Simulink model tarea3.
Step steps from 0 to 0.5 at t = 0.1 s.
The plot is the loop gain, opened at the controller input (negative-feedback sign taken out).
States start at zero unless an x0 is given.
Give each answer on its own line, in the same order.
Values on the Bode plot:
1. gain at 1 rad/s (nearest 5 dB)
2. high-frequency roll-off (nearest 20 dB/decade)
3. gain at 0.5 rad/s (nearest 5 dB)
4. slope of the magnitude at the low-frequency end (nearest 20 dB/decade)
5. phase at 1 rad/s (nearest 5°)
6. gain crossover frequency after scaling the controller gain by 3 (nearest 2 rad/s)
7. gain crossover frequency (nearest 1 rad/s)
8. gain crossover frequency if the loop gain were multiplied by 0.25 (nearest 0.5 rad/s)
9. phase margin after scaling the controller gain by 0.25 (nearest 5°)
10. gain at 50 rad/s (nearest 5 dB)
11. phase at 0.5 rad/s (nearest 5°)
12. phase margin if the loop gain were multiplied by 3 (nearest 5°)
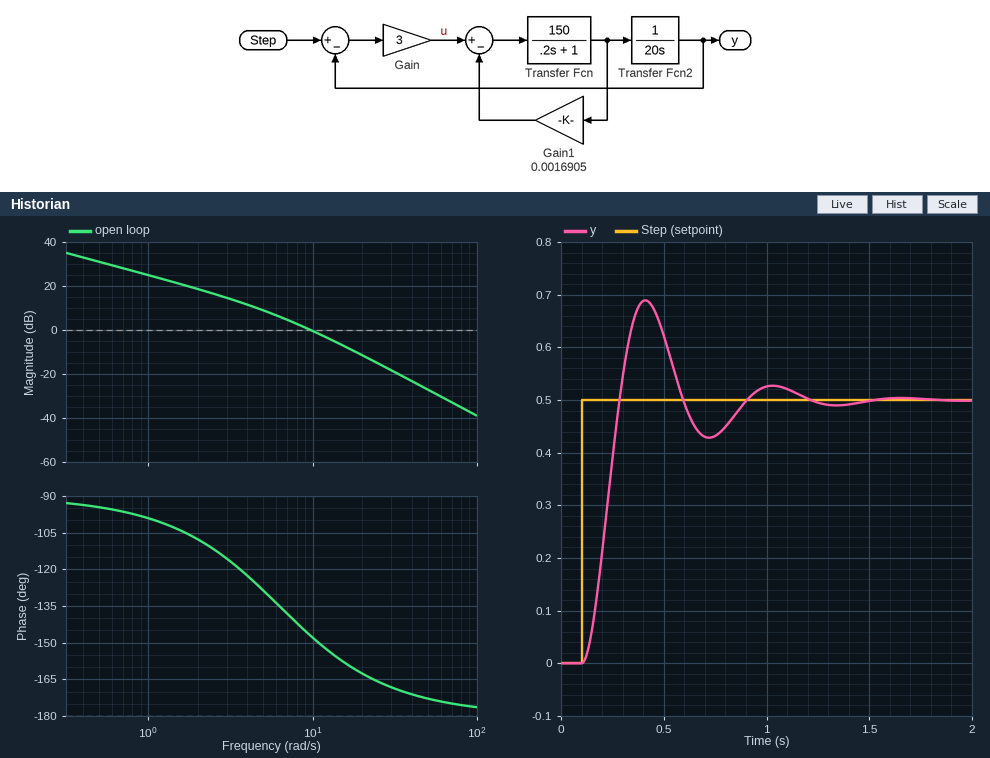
25 dB
-40 dB/decade
30 dB
-20 dB/decade
-100°
18 rad/s
10 rad/s
4.0 rad/s
60°
-25 dB
-95°
20°
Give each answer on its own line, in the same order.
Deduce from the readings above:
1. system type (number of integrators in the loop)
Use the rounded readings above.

1
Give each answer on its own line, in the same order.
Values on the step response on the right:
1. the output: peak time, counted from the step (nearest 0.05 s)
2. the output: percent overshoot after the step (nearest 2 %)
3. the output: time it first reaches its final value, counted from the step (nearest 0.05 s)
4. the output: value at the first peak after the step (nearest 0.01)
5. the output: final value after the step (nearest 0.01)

0.30 s
38 %
0.20 s
0.69
0.50
